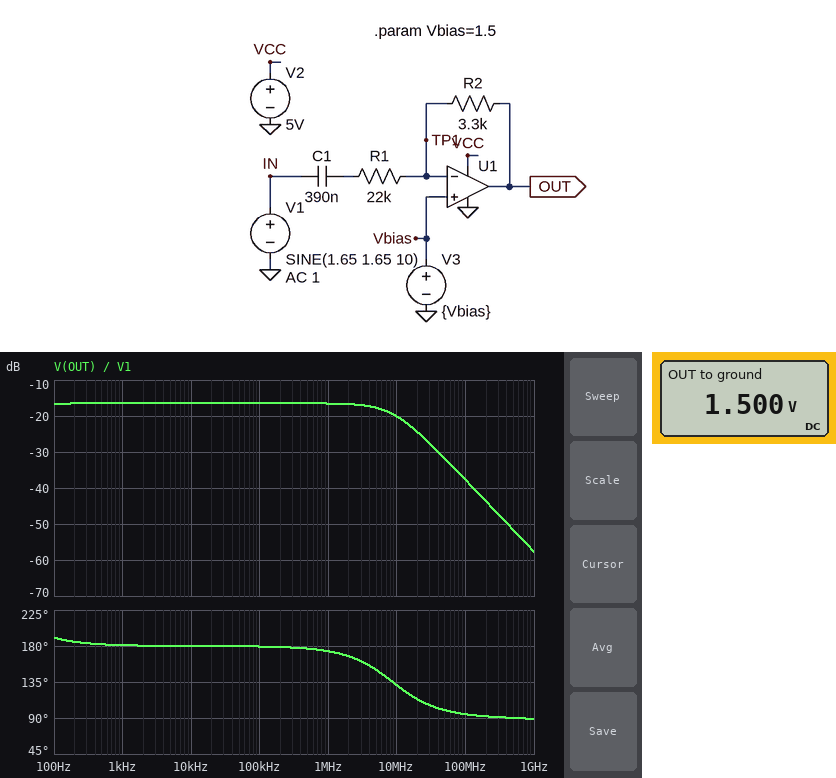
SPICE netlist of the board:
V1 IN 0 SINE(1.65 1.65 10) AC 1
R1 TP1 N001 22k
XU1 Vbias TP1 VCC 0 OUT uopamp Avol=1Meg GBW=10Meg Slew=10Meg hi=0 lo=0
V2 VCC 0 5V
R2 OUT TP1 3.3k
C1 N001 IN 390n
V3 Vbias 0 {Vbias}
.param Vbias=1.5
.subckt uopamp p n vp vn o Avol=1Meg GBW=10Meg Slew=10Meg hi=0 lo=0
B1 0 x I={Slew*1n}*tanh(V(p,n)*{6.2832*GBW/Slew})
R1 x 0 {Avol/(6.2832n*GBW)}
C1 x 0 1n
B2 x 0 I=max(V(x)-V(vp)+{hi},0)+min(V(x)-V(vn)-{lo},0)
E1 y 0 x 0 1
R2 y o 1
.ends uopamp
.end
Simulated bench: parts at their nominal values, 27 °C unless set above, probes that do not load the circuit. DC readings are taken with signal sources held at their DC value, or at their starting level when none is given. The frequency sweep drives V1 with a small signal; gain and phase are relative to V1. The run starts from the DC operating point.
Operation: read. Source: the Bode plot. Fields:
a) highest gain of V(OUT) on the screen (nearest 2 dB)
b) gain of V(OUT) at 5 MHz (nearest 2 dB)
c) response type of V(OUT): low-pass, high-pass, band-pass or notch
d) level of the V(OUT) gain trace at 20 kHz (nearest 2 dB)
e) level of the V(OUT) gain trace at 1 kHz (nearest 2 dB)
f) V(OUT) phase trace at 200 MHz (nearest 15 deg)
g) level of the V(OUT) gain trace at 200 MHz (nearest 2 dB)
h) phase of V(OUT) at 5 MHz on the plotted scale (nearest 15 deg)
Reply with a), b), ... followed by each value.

a) -16 dB
b) -18 dB
c) low-pass
d) -16 dB
e) -16 dB
f) 90 deg
g) -44 dB
h) 150 deg
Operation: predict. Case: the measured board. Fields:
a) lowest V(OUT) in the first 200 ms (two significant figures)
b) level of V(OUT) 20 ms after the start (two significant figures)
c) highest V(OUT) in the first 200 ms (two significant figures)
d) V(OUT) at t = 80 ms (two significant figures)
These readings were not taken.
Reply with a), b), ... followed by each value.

a) 1.4 V
b) 1.4 V
c) 1.6 V
d) 1.5 V
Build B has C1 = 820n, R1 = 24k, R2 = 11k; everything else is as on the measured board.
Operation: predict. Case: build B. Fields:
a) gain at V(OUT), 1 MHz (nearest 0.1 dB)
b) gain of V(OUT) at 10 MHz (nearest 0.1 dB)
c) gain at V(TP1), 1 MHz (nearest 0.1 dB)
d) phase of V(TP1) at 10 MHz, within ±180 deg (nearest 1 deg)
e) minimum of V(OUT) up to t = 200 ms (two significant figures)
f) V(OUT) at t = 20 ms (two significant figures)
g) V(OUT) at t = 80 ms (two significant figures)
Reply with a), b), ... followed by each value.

a) -6.9 dB
b) -11.7 dB
c) -26.9 dB
d) 34 deg
e) 910 mV
f) 1.1 V
g) 1.8 V
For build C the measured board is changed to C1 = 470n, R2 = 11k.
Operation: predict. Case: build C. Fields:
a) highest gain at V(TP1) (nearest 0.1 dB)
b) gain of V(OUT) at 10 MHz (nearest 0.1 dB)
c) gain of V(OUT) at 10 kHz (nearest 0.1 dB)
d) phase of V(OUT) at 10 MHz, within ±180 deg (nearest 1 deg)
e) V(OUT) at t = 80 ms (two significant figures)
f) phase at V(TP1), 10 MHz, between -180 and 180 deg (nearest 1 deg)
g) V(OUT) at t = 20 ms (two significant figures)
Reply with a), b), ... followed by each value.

a) -9.5 dB
b) -11.1 dB
c) -6.0 dB
d) 124 deg
e) 1.6 V
f) 34 deg
g) 1.2 V
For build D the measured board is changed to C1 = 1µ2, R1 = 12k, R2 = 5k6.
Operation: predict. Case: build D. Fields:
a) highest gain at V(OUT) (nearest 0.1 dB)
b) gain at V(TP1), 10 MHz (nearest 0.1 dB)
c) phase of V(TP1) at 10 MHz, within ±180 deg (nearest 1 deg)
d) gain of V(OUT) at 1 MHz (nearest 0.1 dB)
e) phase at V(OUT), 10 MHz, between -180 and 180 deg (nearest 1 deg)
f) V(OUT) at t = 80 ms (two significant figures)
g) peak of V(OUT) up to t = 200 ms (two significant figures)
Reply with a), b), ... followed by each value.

a) -6.6 dB
b) -11.6 dB
c) 34 deg
d) -6.7 dB
e) 124 deg
f) 1.7 V
g) 2.0 V
